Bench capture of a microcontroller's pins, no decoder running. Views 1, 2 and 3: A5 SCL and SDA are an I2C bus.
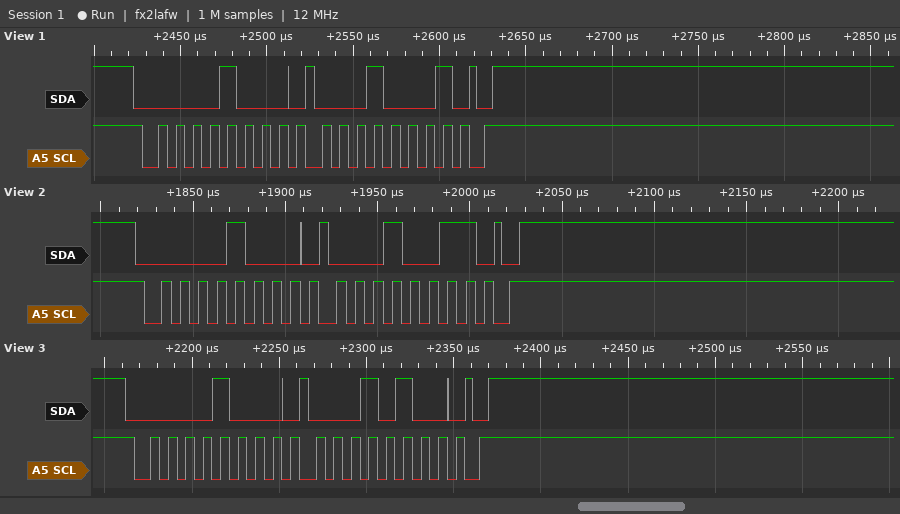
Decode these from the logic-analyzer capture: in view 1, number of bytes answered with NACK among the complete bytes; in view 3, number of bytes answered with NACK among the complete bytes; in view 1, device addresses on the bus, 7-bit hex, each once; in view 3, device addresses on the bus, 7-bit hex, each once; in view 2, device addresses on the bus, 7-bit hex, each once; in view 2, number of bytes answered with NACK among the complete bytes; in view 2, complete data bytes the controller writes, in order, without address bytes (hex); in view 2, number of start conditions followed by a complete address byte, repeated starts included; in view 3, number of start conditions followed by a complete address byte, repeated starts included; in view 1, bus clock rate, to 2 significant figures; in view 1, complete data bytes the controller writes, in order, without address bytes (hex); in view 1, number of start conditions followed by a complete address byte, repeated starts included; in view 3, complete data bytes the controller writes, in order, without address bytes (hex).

0
0
0x04
0x04
0x04
0
13
1
1
100 kHz
11
1
14
